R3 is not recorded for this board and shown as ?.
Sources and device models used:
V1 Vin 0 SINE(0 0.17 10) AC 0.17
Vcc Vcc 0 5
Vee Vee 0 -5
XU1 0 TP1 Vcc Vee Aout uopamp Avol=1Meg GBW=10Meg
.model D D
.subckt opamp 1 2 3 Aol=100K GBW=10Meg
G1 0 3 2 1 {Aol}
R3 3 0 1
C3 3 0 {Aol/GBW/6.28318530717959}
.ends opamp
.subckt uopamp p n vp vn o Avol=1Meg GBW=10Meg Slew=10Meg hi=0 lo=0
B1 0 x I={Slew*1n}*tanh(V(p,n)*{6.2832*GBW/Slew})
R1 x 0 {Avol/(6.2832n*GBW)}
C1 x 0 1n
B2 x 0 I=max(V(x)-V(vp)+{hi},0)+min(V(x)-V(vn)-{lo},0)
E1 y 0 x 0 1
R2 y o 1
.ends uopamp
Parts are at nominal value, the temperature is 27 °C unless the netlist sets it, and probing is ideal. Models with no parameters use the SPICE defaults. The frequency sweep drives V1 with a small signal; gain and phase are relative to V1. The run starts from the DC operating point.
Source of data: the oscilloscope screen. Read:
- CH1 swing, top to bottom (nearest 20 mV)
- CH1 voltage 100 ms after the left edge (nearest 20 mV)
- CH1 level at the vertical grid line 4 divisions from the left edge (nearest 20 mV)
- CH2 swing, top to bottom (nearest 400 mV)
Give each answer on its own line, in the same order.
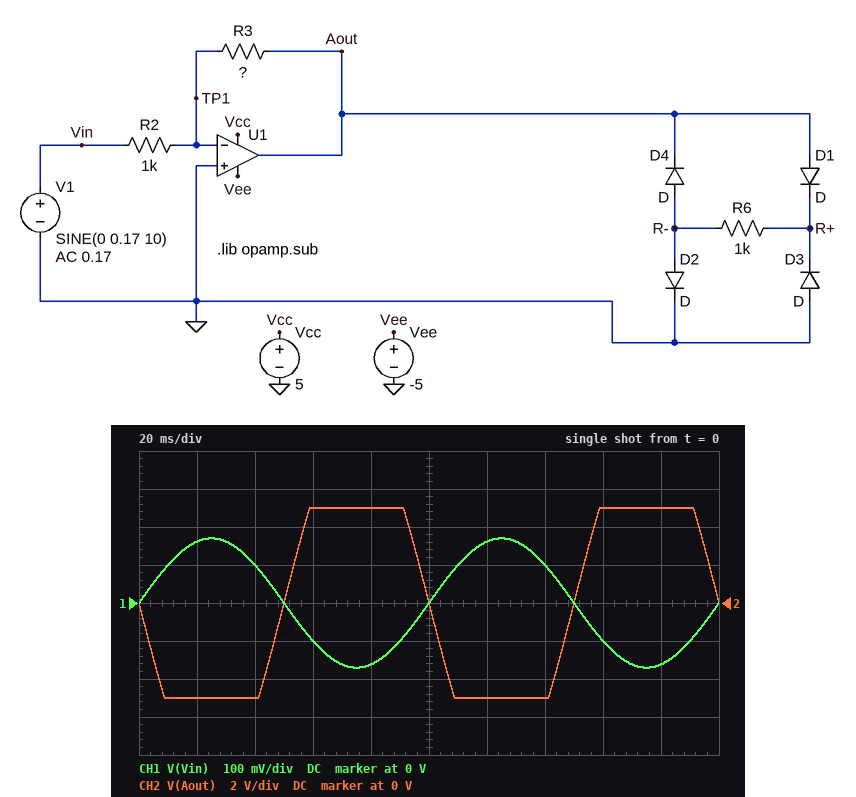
340 mV
0 V
-160 mV
10.0 V
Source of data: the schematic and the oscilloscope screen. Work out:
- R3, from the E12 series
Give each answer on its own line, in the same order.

56 kΩ
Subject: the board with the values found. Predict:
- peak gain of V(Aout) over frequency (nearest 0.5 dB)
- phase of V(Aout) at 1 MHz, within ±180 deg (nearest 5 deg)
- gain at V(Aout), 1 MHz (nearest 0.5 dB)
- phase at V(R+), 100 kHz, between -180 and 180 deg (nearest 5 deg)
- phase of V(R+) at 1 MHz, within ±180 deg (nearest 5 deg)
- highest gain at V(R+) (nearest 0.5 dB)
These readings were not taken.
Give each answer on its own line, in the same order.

35.0 dB
100 deg
19.5 dB
150 deg
100 deg
29.0 dB
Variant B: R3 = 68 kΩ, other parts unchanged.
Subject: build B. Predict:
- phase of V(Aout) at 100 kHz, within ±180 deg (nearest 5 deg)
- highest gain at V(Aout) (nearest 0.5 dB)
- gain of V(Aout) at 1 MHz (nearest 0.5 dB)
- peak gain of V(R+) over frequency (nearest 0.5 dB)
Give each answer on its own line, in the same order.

145 deg
36.5 dB
20.0 dB
30.5 dB
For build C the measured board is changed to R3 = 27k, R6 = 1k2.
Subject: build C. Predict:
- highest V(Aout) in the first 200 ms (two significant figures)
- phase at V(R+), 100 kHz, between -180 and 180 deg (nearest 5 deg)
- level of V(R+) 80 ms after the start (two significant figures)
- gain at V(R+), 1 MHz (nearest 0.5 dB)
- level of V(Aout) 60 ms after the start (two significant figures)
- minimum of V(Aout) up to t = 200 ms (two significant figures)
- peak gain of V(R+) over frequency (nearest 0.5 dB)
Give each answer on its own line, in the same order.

4.6 V
165 deg
3.7 V
13.0 dB
2.7 V
-4.6 V
22.5 dB
